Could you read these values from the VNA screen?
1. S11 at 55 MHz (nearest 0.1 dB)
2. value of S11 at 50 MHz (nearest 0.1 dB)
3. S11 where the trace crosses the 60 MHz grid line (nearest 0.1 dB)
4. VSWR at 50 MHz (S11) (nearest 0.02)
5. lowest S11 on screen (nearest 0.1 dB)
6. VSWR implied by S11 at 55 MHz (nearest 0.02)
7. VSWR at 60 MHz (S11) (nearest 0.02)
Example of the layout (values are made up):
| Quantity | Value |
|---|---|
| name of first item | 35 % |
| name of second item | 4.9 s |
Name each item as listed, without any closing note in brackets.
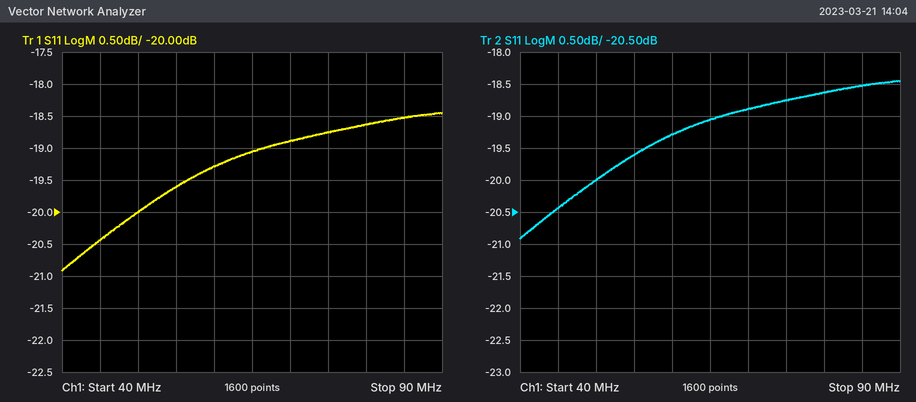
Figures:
| Quantity | Value |
|---|---|
| S11 at 55 MHz | -19.6 dB |
| value of S11 at 50 MHz | -20.0 dB |
| S11 where the trace crosses the 60 MHz grid line | -19.3 dB |
| VSWR at 50 MHz (S11) | 1.22 |
| lowest S11 on screen | -20.9 dB |
| VSWR implied by S11 at 55 MHz | 1.24 |
| VSWR at 60 MHz (S11) | 1.24 |
